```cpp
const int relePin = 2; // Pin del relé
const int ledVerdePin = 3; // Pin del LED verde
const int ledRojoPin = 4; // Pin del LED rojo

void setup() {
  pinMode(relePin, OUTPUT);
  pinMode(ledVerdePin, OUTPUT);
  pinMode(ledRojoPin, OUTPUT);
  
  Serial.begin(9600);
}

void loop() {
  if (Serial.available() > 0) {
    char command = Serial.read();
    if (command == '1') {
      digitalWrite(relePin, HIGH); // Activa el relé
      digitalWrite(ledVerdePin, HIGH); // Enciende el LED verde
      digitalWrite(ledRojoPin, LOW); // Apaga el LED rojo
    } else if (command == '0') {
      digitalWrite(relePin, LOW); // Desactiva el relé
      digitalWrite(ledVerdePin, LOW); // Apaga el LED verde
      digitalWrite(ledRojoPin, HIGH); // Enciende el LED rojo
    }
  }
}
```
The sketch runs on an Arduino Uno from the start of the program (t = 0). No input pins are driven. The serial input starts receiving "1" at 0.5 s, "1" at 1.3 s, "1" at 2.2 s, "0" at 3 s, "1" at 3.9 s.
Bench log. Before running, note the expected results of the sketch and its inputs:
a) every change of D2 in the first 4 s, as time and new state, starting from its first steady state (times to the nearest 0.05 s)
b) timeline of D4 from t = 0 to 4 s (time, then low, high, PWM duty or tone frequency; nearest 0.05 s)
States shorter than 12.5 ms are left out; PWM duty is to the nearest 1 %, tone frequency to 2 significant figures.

0 s low; 0.5 s high; 3 s low; 3.9 s high
0 s low; 3 s high; 3.9 s low
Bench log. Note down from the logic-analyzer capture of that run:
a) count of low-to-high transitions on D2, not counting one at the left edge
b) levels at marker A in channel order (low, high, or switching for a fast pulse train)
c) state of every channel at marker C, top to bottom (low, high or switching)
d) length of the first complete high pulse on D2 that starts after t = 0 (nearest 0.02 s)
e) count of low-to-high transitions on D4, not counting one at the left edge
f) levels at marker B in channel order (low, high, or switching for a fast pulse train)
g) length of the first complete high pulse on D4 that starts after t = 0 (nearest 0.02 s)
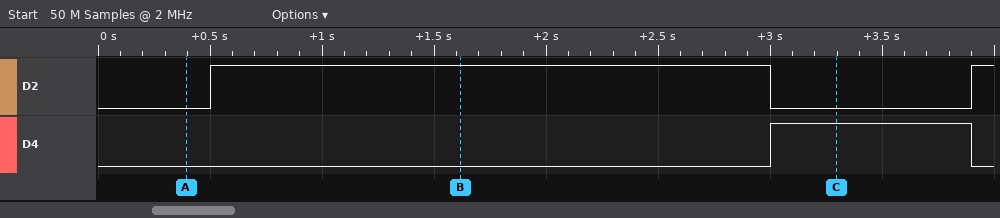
2
D2 low, D4 low
D2 low, D4 high
2.50 s
1
D2 high, D4 low
0.90 s
